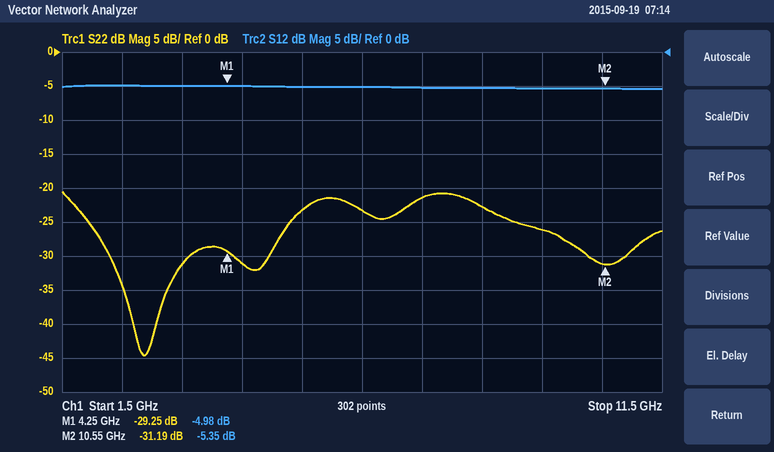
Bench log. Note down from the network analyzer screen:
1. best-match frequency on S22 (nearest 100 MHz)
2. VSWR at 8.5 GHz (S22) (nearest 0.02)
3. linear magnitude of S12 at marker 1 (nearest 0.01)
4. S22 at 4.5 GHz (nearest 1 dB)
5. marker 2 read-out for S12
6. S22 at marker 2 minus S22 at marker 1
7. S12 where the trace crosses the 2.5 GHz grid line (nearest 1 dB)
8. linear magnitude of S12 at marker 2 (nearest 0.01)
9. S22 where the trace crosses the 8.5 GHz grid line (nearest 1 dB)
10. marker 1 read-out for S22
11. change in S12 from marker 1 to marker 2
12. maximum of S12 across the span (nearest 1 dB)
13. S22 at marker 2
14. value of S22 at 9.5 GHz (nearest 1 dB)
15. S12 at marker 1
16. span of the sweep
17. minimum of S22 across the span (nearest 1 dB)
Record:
2.9 GHz
1.16
0.56
-31 dB
-5.35 dB
-1.94 dB
-5 dB
0.54
-23 dB
-29.25 dB
-0.37 dB
-5 dB
-31.19 dB
-26 dB
-4.98 dB
10 GHz
-45 dB
